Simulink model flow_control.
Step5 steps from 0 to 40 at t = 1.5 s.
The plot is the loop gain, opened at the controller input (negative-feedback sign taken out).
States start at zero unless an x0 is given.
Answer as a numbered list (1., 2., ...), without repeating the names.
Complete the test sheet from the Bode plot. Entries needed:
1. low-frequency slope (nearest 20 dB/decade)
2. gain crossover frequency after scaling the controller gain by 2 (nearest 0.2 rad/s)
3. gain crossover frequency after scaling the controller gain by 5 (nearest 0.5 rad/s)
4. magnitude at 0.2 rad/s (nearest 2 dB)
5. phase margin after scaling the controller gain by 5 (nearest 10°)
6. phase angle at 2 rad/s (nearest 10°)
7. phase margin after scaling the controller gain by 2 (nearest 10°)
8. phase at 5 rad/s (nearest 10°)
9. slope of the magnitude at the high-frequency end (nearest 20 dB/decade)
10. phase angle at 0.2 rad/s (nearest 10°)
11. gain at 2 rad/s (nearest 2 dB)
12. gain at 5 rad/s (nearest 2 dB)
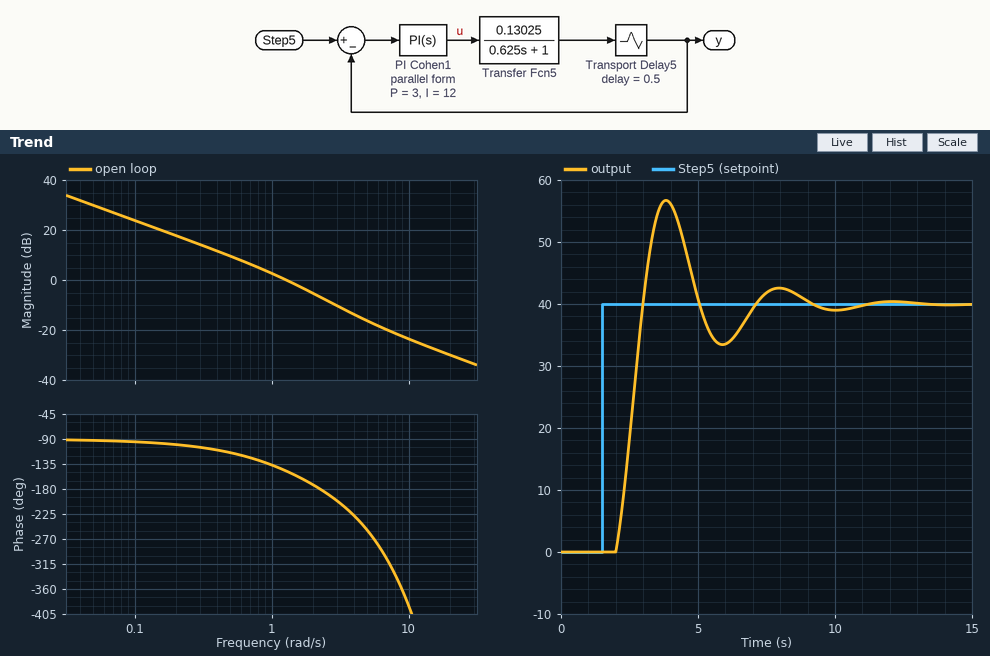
1. -20 dB/decade
2. 2.2 rad/s
3. 4.0 rad/s
4. 18 dB
5. -50°
6. -170°
7. 0°
8. -250°
9. -20 dB/decade
10. -100°
11. -6 dB
12. -16 dB
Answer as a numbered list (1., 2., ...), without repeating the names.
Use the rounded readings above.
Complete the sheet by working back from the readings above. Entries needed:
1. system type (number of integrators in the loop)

1. 1
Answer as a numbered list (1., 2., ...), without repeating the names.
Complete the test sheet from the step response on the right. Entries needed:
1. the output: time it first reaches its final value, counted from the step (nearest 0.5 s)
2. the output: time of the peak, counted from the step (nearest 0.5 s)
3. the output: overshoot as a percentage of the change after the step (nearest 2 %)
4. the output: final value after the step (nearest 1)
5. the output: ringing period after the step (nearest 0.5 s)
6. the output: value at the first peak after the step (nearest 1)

1. 1.5 s
2. 2.5 s
3. 42 %
4. 40
5. 4.0 s
6. 57
